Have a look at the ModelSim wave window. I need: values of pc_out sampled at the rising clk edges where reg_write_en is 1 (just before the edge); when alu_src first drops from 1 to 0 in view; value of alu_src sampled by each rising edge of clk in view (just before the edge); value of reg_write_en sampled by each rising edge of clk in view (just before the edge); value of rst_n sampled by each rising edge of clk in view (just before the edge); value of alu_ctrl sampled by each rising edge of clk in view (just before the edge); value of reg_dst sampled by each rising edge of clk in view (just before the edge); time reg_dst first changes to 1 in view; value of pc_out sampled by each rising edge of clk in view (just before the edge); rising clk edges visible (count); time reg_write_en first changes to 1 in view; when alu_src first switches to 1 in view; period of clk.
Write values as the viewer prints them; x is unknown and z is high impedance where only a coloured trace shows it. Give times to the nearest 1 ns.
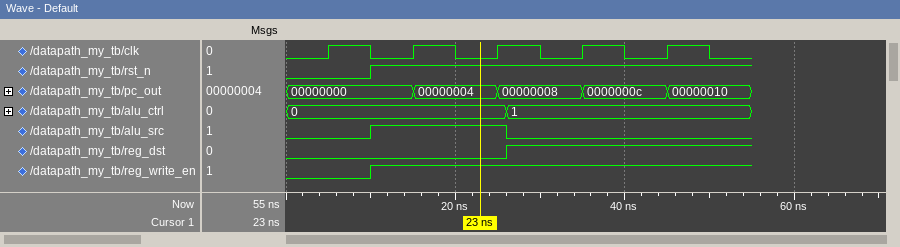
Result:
00000000, 00000004, 00000008, 0000000c
26 ns
0 1 1 0 0
0 1 1 1 1
0 1 1 1 1
0, 0, 0, 1, 1
0 0 0 1 1
26 ns
00000000, 00000000, 00000004, 00000008, 0000000c
5
10 ns
10 ns
10 ns
